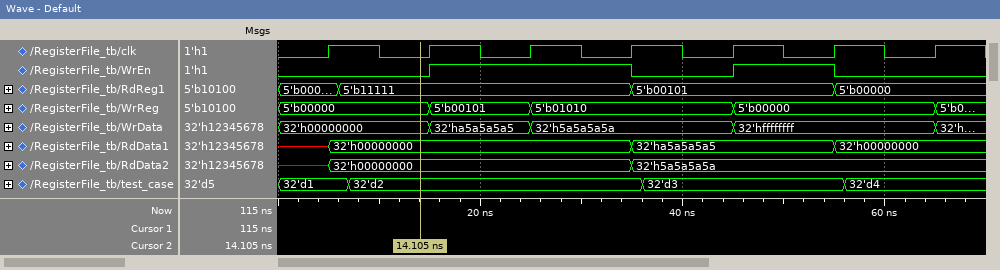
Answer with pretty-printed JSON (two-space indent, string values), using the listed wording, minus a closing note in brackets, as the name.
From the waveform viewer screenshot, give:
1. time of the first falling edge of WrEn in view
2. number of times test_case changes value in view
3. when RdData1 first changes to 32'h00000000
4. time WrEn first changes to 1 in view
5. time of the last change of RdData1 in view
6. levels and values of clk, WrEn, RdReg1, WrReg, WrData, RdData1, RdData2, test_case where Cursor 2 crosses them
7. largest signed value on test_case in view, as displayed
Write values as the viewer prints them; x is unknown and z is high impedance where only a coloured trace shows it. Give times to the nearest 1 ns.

{
  "time of the first falling edge of WrEn in view": "35 ns",
  "number of times test_case changes value in view": "3",
  "when RdData1 first changes to 32'h00000000": "5 ns",
  "time WrEn first changes to 1 in view": "15 ns",
  "time of the last change of RdData1 in view": "55 ns",
  "levels and values of clk, WrEn, RdReg1, WrReg, WrData, RdData1, RdData2, test_case where Cursor 2 crosses them": "clk=0, WrEn=0, RdReg1=5'b11111, WrReg=5'b00000, WrData=32'h00000000, RdData1=32'h00000000, RdData2=32'h00000000, test_case=32'd2",
  "largest signed value on test_case in view, as displayed": "32'd4"
}
